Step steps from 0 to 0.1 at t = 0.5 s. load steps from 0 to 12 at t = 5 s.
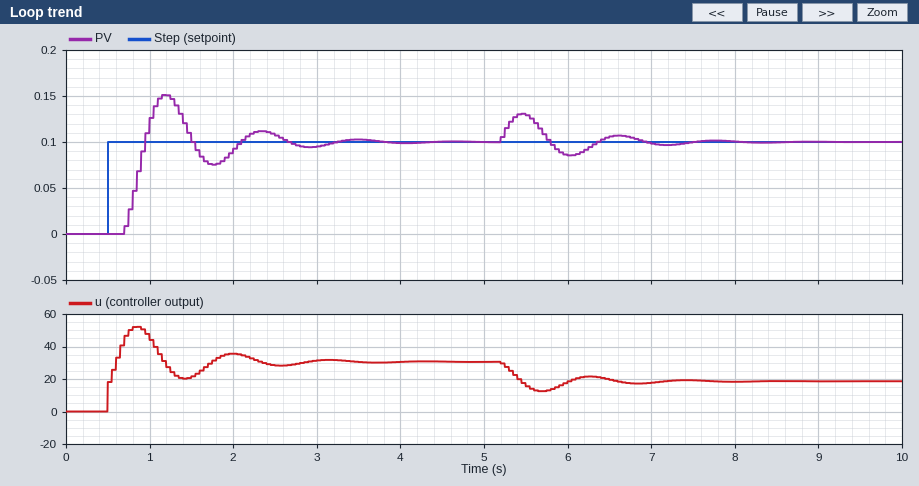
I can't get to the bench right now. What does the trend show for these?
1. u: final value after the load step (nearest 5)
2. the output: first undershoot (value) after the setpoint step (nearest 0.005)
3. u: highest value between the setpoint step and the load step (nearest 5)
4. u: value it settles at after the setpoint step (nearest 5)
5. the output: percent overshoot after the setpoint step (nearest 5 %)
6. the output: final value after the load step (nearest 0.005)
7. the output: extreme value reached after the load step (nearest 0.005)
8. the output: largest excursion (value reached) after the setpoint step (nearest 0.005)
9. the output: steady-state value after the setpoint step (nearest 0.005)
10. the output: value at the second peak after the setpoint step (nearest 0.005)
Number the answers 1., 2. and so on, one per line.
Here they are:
1. 20
2. 0.075
3. 50
4. 30
5. 50 %
6. 0.100
7. 0.130
8. 0.150
9. 0.100
10. 0.110
